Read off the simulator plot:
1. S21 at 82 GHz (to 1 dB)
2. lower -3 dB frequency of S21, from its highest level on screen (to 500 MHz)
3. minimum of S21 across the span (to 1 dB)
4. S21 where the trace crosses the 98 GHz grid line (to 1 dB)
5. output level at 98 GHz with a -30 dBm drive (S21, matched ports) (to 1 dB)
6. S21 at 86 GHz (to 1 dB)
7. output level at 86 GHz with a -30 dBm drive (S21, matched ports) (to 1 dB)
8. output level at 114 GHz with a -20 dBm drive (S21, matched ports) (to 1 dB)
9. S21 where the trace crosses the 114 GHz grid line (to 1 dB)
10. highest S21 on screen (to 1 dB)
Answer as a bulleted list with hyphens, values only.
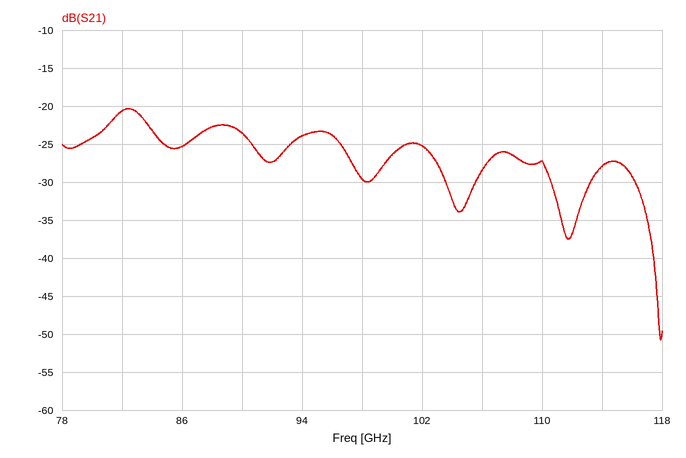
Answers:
- -21 dB
- 80.5 GHz
- -51 dB
- -30 dB
- -60 dBm
- -25 dB
- -55 dBm
- -48 dBm
- -28 dB
- -20 dB
